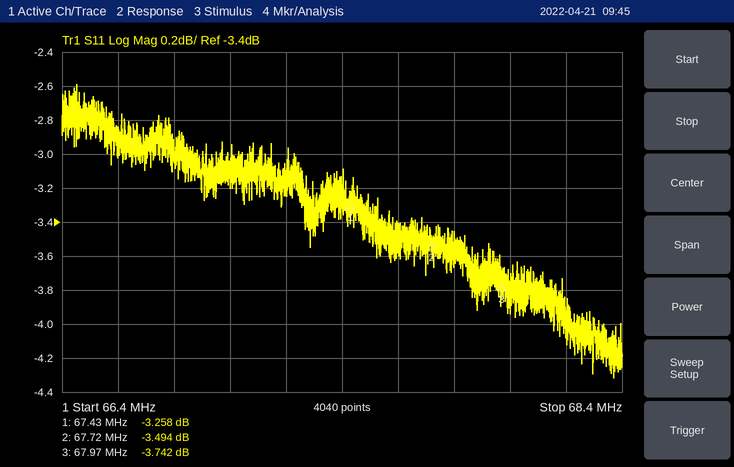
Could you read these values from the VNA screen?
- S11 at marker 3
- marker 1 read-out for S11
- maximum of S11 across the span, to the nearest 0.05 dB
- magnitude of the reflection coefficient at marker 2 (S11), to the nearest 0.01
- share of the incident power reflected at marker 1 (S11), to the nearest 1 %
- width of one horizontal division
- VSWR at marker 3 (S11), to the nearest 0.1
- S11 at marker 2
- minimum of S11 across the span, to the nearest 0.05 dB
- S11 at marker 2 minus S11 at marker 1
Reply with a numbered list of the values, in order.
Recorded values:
1. -3.742 dB
2. -3.258 dB
3. -2.60 dB
4. 0.67
5. 47 %
6. 200 kHz
7. 4.7
8. -3.494 dB
9. -4.30 dB
10. -0.236 dB
